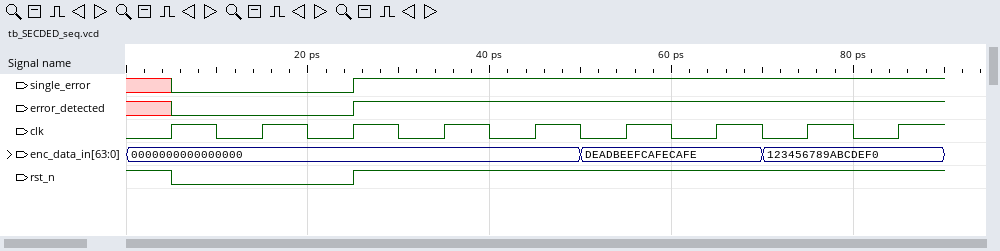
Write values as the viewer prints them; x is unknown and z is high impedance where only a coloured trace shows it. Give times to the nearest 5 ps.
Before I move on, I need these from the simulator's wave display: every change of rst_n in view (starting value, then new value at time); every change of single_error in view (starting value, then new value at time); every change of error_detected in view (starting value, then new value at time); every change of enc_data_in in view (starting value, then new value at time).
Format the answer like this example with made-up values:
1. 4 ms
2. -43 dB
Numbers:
1. 1, 0 at 5 ps, 1 at 25 ps
2. x, 0 at 5 ps, 1 at 25 ps
3. x, 0 at 5 ps, 1 at 25 ps
4. 0000000000000000, DEADBEEFCAFECAFE at 50 ps, 123456789ABCDEF0 at 70 ps
